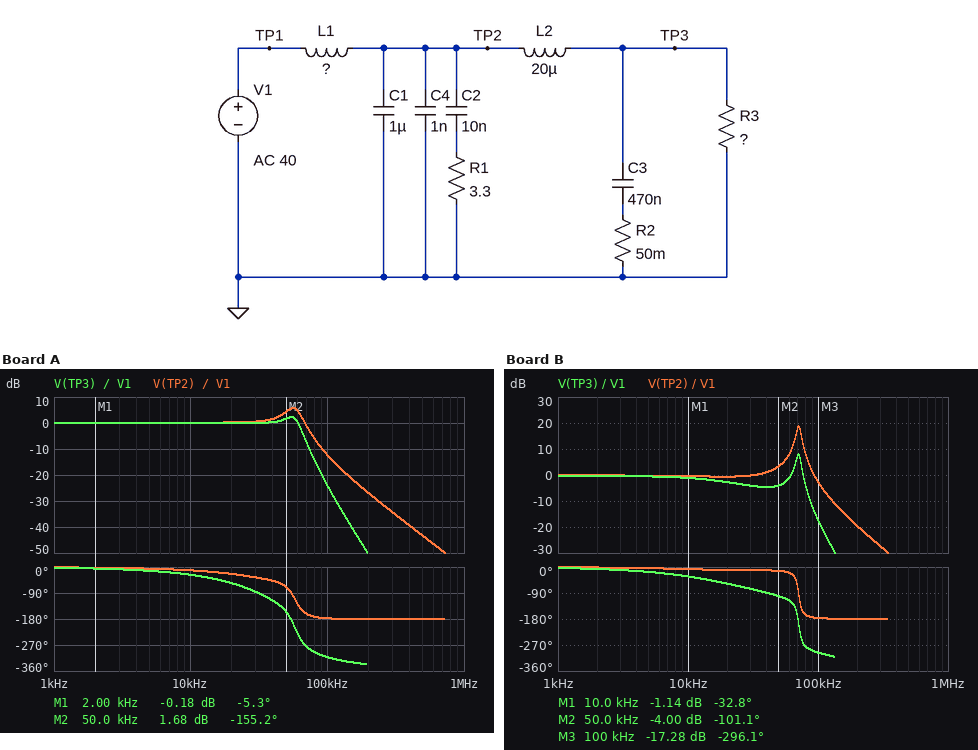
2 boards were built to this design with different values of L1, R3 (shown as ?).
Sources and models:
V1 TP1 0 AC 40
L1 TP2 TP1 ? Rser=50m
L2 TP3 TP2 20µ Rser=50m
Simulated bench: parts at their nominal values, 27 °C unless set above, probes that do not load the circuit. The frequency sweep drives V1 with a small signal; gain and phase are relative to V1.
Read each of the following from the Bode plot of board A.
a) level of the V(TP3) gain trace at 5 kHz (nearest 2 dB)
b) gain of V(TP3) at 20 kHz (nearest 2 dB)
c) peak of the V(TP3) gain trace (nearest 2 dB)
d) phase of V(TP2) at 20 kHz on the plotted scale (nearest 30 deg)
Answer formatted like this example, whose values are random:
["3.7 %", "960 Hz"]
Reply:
["0 dB", "0 dB", "2 dB", "-30 deg"]
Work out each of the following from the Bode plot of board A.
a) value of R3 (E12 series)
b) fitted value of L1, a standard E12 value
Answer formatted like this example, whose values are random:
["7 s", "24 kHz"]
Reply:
["4.7 Ω", "15 µH"]
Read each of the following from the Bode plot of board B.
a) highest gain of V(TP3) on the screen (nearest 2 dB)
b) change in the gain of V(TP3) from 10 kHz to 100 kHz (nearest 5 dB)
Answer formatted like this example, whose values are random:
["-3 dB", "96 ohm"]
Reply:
["8 dB", "-15 dB"]
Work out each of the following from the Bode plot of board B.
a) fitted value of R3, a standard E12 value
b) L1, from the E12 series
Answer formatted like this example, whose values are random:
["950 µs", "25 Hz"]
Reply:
["2.7 Ω", "6.8 µH"]
